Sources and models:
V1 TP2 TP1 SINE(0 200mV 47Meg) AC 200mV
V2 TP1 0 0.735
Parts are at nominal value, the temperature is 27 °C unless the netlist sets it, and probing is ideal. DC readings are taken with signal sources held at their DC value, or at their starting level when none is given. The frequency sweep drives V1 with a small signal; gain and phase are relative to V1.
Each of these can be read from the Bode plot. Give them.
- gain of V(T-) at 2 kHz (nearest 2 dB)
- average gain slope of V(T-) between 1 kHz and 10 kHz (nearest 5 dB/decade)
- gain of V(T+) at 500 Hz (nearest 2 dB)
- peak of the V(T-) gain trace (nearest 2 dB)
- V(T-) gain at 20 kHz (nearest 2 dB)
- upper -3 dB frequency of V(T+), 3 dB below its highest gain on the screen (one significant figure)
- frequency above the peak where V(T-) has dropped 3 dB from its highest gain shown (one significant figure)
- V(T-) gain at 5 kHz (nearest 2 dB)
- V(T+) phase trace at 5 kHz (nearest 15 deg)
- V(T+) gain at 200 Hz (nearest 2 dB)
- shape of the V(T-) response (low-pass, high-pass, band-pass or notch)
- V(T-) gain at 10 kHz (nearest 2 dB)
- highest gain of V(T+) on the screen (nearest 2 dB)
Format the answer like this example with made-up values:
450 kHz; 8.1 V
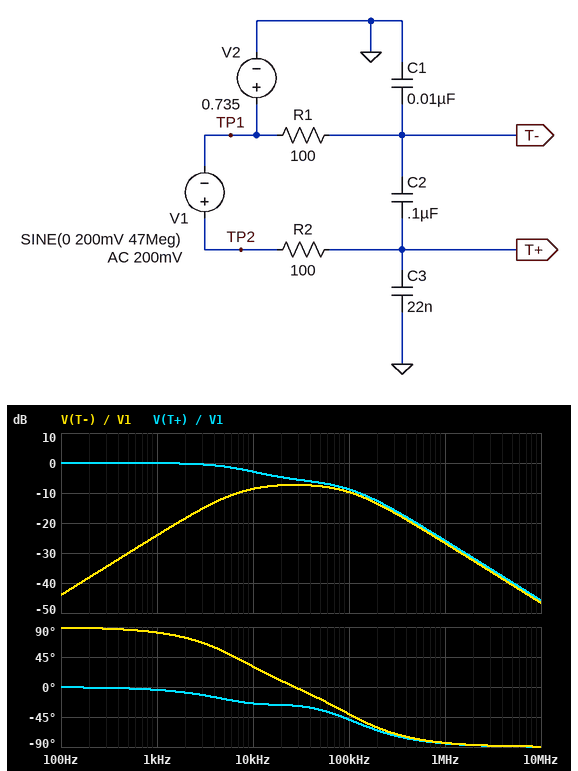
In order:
-18 dB; 15 dB/decade; 0 dB; -8 dB; -8 dB; 10 kHz; 100 kHz; -12 dB; -15 deg; 0 dB; band-pass; -8 dB; 0 dB
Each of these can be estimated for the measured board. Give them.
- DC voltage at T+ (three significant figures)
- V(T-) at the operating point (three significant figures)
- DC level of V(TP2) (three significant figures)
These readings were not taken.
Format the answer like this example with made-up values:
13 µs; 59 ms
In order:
735 mV; 735 mV; 735 mV
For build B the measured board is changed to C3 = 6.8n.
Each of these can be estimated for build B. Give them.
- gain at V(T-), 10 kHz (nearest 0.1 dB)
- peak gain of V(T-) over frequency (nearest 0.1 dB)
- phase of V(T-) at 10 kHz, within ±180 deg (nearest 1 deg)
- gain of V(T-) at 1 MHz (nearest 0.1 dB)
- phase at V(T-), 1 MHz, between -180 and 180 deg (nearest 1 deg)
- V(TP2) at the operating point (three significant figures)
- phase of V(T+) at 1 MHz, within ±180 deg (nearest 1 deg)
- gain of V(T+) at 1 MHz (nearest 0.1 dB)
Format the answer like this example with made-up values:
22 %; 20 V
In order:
-8.4 dB; -6.7 dB; 34 deg; -21.0 dB; -79 deg; 735 mV; -80 deg; -20.1 dB
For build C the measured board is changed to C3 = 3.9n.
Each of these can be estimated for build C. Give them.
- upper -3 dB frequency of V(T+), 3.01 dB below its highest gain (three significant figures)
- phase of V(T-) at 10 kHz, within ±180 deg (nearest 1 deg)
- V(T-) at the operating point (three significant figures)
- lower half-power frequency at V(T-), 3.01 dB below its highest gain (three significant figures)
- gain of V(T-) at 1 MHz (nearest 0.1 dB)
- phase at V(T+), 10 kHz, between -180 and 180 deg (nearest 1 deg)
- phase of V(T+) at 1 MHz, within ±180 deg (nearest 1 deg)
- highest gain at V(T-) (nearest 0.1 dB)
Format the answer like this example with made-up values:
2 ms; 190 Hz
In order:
11.6 kHz; 35 deg; 735 mV; 7.22 kHz; -19.3 dB; -20 deg; -77 deg; -6.6 dB
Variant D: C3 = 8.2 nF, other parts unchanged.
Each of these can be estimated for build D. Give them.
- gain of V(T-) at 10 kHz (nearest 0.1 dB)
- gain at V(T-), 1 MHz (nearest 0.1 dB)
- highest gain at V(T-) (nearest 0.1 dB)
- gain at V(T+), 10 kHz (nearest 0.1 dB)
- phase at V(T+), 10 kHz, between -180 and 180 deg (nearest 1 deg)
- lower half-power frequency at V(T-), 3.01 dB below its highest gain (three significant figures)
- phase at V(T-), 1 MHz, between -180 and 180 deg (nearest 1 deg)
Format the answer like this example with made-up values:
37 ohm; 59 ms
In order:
-8.4 dB; -21.7 dB; -6.8 dB; -2.7 dB; -21 deg; 7.02 kHz; -80 deg
